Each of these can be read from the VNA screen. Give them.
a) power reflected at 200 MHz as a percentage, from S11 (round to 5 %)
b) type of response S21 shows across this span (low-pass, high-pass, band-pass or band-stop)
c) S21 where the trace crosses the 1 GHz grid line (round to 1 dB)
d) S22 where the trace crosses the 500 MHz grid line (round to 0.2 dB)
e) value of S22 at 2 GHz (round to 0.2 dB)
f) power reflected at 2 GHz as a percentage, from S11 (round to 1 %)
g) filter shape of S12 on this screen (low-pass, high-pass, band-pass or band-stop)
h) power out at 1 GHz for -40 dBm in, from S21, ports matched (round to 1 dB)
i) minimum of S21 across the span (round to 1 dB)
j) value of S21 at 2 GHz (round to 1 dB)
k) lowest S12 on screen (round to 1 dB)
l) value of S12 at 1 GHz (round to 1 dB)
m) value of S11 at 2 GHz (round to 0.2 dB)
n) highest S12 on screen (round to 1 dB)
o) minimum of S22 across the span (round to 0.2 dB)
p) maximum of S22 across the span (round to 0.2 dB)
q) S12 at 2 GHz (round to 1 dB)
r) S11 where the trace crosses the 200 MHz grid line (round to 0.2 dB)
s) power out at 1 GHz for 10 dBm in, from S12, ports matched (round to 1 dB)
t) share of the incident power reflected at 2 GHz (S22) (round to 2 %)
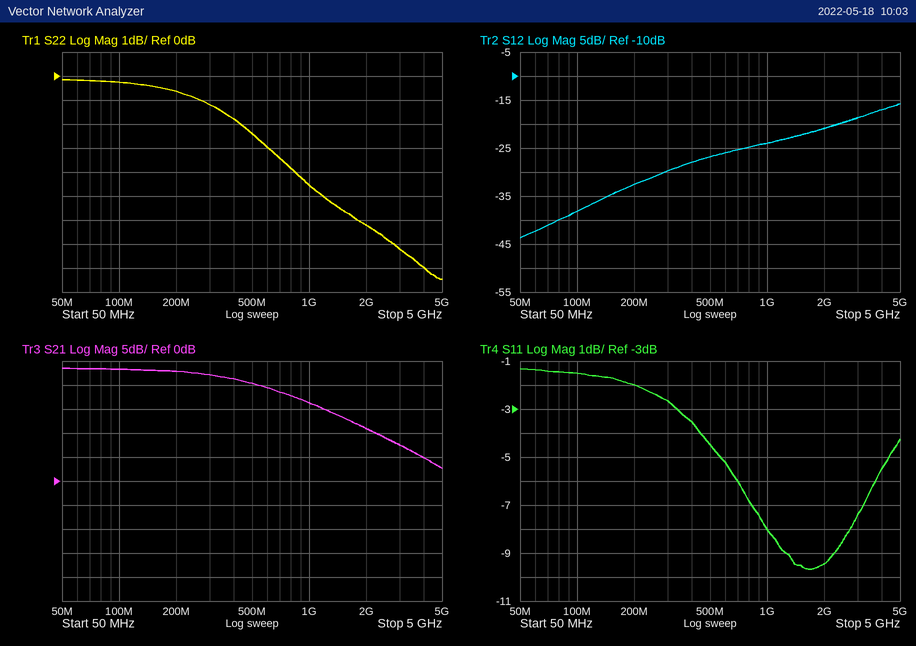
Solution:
65 %
low-pass
16 dB
-2.4 dB
-6.2 dB
11 %
high-pass
-24 dBm
3 dB
11 dB
-44 dB
-24 dB
-9.4 dB
-16 dB
-8.4 dB
-0.2 dB
-21 dB
-2.0 dB
-14 dBm
24 %
